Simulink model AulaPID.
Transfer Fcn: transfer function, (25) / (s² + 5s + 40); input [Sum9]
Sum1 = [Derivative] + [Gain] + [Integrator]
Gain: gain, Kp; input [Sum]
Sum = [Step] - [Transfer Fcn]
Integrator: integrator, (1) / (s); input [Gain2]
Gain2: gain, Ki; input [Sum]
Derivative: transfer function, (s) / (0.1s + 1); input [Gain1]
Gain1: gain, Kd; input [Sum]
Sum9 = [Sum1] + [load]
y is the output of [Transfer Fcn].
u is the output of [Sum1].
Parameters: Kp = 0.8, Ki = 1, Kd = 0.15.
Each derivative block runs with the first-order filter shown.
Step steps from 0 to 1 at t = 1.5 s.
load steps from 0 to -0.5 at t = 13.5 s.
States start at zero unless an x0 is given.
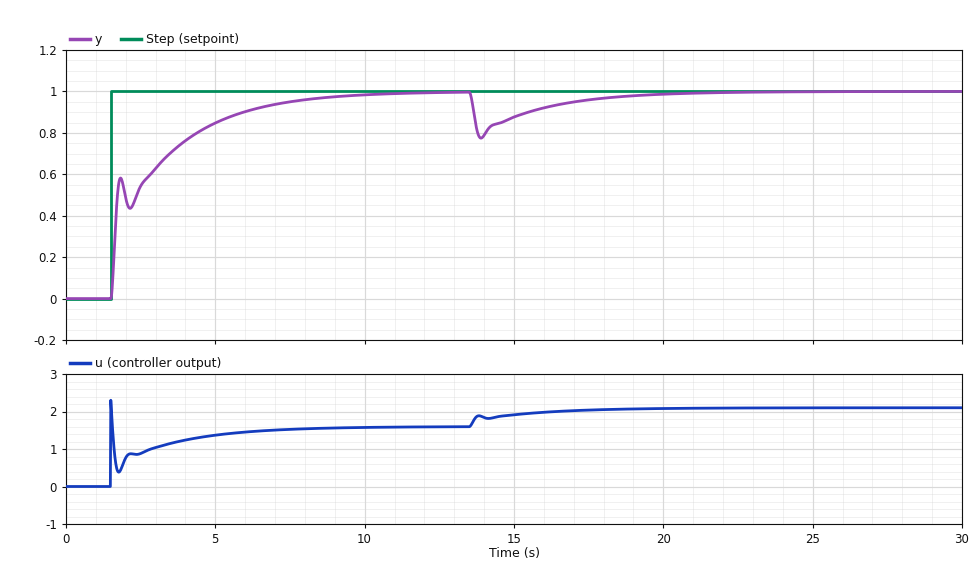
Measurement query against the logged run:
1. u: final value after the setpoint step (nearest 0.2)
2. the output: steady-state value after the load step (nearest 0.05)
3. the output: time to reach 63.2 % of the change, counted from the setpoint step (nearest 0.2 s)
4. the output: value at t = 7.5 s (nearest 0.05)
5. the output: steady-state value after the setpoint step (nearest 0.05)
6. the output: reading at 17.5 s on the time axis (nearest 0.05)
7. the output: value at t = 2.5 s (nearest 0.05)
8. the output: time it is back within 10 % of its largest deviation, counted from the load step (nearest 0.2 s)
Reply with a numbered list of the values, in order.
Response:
1. 1.6
2. 1.00
3. 1.6 s
4. 0.95
5. 1.00
6. 0.95
7. 0.55
8. 5.4 s
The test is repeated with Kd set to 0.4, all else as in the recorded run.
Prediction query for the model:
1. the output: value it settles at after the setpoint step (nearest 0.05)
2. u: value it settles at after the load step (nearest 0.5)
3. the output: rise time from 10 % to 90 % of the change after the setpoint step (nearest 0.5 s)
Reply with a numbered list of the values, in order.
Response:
1. 1.00
2. 2.0
3. 4.5 s
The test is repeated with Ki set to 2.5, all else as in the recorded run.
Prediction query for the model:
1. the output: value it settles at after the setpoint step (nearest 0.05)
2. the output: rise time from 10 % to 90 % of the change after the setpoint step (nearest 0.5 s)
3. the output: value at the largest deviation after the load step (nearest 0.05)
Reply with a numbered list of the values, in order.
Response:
1. 1.00
2. 1.5 s
3. 0.80
